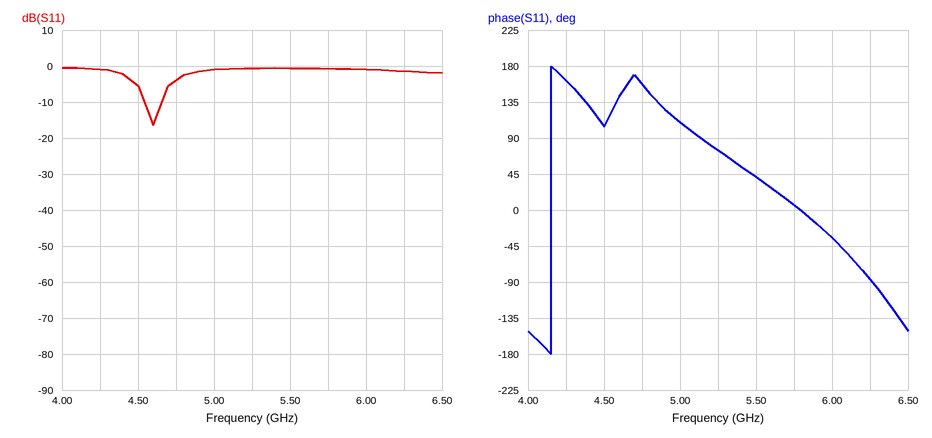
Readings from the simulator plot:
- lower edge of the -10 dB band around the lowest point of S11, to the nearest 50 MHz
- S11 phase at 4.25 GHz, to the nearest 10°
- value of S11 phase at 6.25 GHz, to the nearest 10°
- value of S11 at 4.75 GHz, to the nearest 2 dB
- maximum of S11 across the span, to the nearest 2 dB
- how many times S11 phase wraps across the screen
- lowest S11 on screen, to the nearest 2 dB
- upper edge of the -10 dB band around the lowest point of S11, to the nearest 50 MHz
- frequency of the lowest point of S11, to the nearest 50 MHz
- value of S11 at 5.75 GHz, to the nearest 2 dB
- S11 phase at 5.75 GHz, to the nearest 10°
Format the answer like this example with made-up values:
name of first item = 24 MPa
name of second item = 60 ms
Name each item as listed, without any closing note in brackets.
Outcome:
lower edge of the -10 dB band around the lowest point of S11, to the nearest 50 MHz = 4.55 GHz
S11 phase at 4.25 GHz, to the nearest 10° = 160°
value of S11 phase at 6.25 GHz, to the nearest 10° = -90°
value of S11 at 4.75 GHz, to the nearest 2 dB = -4 dB
maximum of S11 across the span, to the nearest 2 dB = 0 dB
how many times S11 phase wraps across the screen = 1
lowest S11 on screen, to the nearest 2 dB = -16 dB
upper edge of the -10 dB band around the lowest point of S11, to the nearest 50 MHz = 4.65 GHz
frequency of the lowest point of S11, to the nearest 50 MHz = 4.60 GHz
value of S11 at 5.75 GHz, to the nearest 2 dB = 0 dB
S11 phase at 5.75 GHz, to the nearest 10° = 10°
